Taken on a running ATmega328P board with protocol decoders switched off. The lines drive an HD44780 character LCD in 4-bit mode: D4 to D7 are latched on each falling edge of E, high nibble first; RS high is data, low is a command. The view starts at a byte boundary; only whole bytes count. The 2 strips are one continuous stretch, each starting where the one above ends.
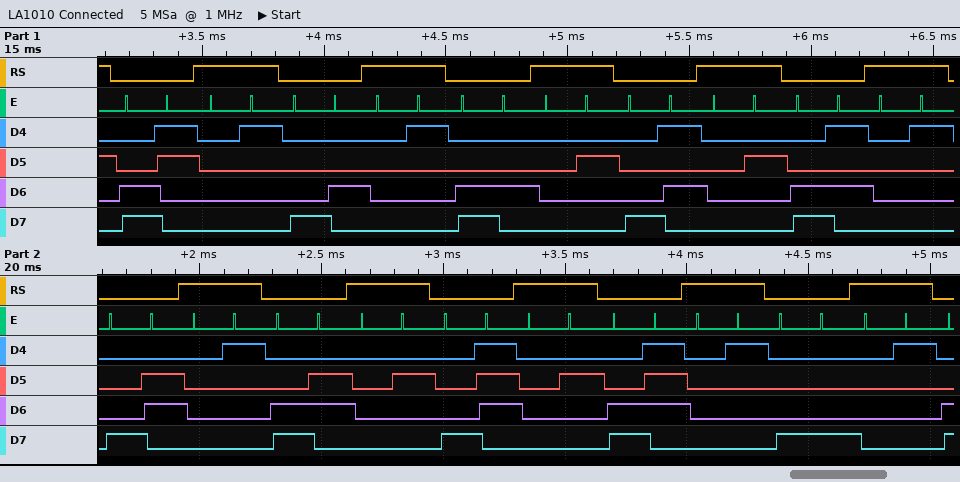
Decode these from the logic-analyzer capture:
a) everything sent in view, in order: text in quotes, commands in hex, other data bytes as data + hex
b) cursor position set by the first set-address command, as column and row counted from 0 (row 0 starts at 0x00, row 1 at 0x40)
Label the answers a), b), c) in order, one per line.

a) 0xC3 data 01 0x84 data 01 0xC4 data 02 0x85 data 02 0xC5 data 01 0x86 data 01 0xC6 data 02 0x87 data 02 0xC7 data 01 0x88 data 01
b) column 3, row 1
